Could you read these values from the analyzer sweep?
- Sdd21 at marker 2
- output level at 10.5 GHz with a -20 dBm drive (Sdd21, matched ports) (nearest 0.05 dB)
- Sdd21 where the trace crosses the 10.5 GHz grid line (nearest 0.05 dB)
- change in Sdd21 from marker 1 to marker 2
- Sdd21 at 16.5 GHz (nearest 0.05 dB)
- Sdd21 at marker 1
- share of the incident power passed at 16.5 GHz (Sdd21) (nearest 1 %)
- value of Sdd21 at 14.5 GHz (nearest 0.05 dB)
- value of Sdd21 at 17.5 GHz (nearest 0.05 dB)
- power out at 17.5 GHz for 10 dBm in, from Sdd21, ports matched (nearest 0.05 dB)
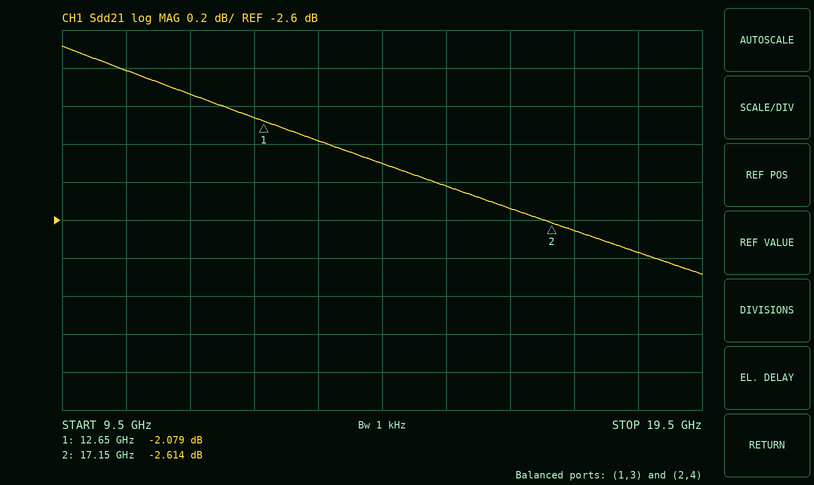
-2.614 dB
-21.80 dBm
-1.80 dB
-0.535 dB
-2.55 dB
-2.079 dB
56 %
-2.30 dB
-2.65 dB
7.35 dBm
